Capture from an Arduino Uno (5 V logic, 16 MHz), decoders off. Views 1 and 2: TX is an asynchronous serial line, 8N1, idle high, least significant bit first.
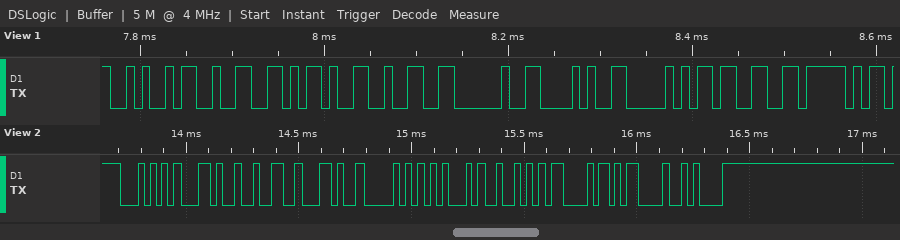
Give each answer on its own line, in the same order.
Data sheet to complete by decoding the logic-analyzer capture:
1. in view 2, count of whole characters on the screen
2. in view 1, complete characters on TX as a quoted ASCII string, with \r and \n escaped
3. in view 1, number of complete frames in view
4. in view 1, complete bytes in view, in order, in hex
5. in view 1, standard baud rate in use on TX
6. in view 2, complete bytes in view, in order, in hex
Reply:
10
"J2-2 (P3_"
9
4A 32 2D 32 20 28 50 33 5F
115200 baud
0x54 0x2C 0x32 0x2C 0x50 0x45 0x52 0x43 0x0D 0x0A
